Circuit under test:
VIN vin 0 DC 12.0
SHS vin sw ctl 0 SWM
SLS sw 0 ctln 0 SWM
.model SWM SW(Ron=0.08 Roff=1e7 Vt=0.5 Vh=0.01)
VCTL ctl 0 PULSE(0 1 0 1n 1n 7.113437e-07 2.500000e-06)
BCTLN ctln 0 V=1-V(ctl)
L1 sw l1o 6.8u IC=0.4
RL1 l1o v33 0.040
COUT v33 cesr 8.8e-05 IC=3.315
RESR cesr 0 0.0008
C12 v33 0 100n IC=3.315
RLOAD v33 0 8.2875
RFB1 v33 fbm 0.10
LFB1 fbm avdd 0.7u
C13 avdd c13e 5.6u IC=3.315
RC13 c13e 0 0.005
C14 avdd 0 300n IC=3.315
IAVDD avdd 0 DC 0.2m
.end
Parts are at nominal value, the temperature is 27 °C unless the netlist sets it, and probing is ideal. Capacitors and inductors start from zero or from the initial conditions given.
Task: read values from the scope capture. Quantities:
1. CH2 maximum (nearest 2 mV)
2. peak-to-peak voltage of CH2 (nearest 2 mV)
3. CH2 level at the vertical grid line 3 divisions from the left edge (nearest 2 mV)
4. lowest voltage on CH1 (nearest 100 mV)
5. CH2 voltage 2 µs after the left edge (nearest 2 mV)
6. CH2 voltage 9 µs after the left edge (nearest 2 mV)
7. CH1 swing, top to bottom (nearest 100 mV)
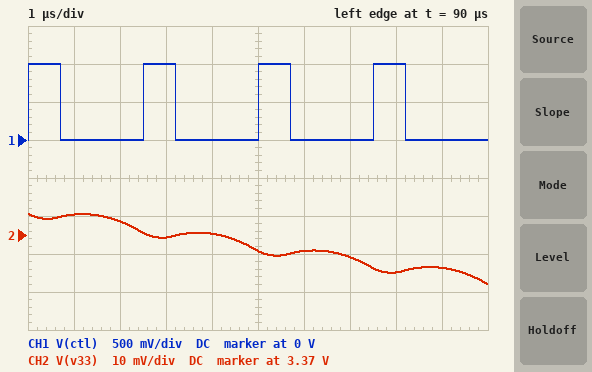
3.376 V
18 mV
3.370 V
0 V
3.374 V
3.362 V
1.0 V
